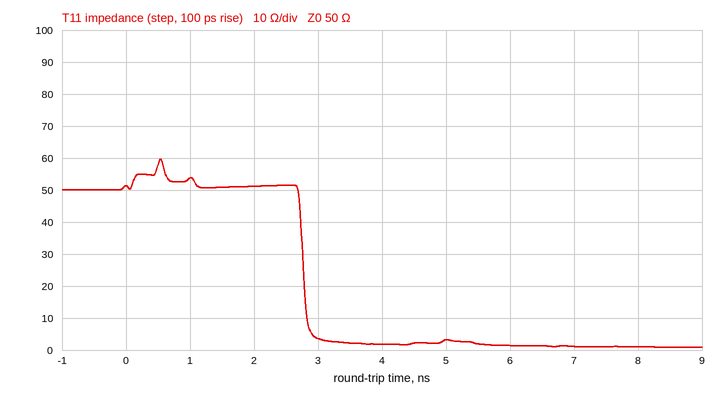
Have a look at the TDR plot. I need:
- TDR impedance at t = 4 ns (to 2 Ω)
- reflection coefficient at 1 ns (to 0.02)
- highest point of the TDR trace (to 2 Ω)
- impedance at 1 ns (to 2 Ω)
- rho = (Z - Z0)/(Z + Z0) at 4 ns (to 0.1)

2 Ω
+0.04
60 Ω
54 Ω
-0.9
